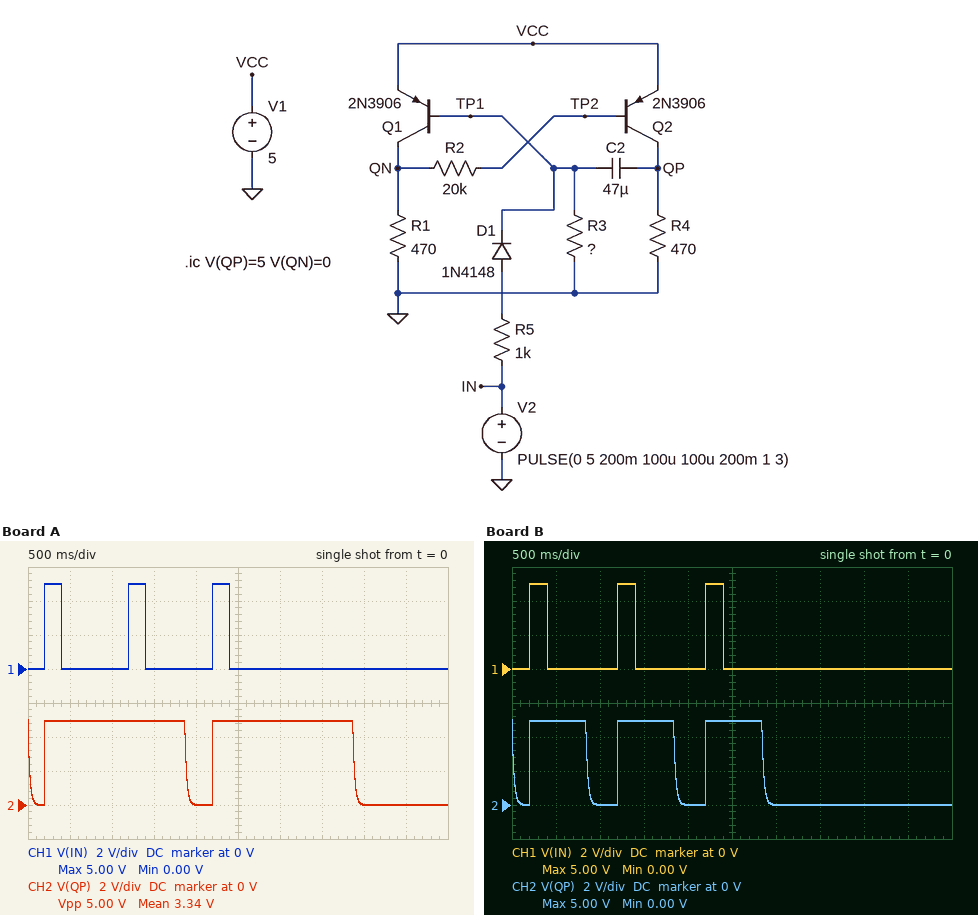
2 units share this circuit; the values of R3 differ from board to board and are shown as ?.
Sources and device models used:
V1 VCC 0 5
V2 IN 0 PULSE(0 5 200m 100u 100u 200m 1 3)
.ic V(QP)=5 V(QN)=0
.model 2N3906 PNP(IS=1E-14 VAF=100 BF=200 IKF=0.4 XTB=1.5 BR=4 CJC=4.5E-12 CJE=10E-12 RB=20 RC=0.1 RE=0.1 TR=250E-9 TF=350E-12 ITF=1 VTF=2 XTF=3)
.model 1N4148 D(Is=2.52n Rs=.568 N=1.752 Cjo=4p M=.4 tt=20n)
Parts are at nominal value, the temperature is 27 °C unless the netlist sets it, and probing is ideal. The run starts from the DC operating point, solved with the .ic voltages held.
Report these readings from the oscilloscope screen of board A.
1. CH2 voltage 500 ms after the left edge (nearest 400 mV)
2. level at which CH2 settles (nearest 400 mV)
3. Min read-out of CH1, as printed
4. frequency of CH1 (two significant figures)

4.8 V
0 V
0.00 V
1.0 Hz
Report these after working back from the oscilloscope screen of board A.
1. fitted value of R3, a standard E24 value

47 kΩ
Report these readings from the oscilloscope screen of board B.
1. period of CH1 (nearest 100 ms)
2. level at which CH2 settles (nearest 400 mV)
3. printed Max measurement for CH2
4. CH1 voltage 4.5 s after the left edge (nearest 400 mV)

1.0 s
0 V
5.00 V
0 V
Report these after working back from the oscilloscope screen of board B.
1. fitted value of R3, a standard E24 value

18 kΩ
